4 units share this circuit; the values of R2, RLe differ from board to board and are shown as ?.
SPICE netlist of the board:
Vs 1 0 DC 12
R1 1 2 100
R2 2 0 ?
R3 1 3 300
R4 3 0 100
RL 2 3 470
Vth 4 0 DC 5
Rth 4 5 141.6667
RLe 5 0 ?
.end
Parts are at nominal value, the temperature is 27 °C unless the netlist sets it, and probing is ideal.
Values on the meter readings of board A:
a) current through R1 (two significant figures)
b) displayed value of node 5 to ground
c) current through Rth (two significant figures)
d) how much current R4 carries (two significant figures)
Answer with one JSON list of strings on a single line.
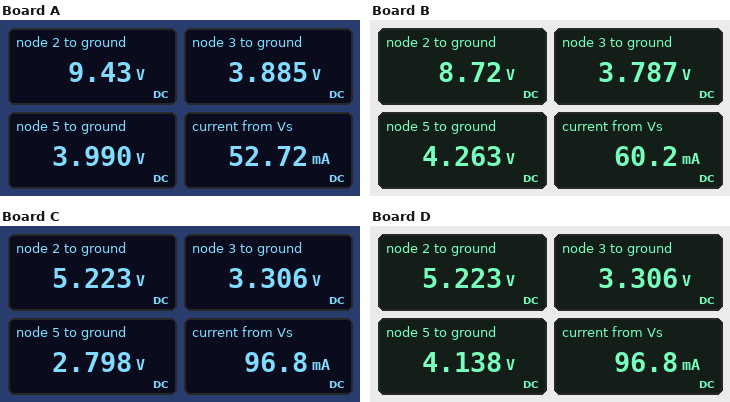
["26 mA", "3.990 V", "7.1 mA", "39 mA"]
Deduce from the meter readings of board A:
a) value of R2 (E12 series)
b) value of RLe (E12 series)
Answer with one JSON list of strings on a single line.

["680 Ω", "560 Ω"]
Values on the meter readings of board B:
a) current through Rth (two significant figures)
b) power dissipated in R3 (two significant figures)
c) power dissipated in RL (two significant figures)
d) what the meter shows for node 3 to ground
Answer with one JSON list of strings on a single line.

["5.2 mA", "220 mW", "52 mW", "3.787 V"]
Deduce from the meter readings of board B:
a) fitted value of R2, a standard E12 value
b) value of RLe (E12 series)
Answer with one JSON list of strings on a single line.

["390 Ω", "820 Ω"]
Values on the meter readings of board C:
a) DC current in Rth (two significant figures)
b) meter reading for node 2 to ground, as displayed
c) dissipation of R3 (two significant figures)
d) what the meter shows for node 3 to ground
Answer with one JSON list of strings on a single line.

["16 mA", "5.223 V", "250 mW", "3.306 V"]
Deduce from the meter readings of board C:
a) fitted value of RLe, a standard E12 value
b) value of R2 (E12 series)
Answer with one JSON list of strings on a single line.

["180 Ω", "82 Ω"]
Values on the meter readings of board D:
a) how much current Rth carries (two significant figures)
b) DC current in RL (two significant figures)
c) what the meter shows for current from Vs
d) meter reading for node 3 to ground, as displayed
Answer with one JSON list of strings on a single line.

["6.1 mA", "4.1 mA", "96.8 mA", "3.306 V"]
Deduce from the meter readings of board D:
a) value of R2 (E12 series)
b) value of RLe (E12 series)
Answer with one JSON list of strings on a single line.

["82 Ω", "680 Ω"]
